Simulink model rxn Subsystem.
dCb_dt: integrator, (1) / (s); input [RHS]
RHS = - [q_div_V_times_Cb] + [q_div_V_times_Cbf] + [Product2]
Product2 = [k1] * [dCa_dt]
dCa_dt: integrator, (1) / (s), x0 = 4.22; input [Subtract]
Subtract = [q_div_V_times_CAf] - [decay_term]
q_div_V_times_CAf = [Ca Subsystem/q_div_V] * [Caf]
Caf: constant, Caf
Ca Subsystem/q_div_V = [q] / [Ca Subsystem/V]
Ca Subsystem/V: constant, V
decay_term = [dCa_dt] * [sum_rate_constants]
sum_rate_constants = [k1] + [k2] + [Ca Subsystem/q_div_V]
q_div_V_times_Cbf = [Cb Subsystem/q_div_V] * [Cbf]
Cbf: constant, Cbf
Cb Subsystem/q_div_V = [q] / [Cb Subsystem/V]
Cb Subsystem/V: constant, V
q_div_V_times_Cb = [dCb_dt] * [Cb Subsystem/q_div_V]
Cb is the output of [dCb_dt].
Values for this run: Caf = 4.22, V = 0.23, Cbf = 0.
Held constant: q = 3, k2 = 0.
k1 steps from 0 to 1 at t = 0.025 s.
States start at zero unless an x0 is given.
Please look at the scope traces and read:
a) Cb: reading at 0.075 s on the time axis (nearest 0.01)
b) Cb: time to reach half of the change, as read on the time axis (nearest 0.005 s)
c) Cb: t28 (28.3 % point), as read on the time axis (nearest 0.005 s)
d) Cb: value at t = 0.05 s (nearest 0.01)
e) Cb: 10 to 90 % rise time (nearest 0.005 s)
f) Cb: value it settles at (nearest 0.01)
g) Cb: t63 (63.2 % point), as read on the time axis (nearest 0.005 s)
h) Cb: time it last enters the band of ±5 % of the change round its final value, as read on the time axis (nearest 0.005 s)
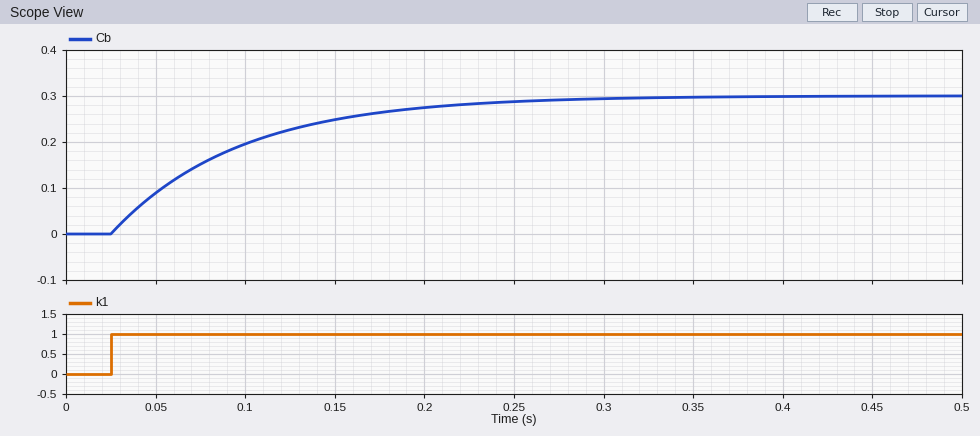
0.15
0.075 s
0.050 s
0.09
0.155 s
0.30
0.095 s
0.240 s
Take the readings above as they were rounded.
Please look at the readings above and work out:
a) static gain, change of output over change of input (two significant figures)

0.30
